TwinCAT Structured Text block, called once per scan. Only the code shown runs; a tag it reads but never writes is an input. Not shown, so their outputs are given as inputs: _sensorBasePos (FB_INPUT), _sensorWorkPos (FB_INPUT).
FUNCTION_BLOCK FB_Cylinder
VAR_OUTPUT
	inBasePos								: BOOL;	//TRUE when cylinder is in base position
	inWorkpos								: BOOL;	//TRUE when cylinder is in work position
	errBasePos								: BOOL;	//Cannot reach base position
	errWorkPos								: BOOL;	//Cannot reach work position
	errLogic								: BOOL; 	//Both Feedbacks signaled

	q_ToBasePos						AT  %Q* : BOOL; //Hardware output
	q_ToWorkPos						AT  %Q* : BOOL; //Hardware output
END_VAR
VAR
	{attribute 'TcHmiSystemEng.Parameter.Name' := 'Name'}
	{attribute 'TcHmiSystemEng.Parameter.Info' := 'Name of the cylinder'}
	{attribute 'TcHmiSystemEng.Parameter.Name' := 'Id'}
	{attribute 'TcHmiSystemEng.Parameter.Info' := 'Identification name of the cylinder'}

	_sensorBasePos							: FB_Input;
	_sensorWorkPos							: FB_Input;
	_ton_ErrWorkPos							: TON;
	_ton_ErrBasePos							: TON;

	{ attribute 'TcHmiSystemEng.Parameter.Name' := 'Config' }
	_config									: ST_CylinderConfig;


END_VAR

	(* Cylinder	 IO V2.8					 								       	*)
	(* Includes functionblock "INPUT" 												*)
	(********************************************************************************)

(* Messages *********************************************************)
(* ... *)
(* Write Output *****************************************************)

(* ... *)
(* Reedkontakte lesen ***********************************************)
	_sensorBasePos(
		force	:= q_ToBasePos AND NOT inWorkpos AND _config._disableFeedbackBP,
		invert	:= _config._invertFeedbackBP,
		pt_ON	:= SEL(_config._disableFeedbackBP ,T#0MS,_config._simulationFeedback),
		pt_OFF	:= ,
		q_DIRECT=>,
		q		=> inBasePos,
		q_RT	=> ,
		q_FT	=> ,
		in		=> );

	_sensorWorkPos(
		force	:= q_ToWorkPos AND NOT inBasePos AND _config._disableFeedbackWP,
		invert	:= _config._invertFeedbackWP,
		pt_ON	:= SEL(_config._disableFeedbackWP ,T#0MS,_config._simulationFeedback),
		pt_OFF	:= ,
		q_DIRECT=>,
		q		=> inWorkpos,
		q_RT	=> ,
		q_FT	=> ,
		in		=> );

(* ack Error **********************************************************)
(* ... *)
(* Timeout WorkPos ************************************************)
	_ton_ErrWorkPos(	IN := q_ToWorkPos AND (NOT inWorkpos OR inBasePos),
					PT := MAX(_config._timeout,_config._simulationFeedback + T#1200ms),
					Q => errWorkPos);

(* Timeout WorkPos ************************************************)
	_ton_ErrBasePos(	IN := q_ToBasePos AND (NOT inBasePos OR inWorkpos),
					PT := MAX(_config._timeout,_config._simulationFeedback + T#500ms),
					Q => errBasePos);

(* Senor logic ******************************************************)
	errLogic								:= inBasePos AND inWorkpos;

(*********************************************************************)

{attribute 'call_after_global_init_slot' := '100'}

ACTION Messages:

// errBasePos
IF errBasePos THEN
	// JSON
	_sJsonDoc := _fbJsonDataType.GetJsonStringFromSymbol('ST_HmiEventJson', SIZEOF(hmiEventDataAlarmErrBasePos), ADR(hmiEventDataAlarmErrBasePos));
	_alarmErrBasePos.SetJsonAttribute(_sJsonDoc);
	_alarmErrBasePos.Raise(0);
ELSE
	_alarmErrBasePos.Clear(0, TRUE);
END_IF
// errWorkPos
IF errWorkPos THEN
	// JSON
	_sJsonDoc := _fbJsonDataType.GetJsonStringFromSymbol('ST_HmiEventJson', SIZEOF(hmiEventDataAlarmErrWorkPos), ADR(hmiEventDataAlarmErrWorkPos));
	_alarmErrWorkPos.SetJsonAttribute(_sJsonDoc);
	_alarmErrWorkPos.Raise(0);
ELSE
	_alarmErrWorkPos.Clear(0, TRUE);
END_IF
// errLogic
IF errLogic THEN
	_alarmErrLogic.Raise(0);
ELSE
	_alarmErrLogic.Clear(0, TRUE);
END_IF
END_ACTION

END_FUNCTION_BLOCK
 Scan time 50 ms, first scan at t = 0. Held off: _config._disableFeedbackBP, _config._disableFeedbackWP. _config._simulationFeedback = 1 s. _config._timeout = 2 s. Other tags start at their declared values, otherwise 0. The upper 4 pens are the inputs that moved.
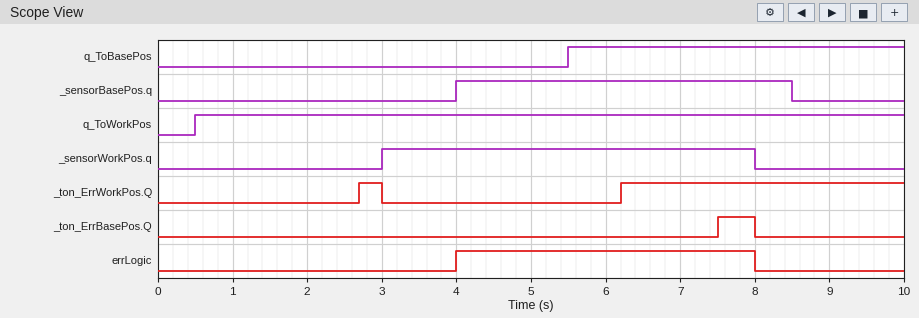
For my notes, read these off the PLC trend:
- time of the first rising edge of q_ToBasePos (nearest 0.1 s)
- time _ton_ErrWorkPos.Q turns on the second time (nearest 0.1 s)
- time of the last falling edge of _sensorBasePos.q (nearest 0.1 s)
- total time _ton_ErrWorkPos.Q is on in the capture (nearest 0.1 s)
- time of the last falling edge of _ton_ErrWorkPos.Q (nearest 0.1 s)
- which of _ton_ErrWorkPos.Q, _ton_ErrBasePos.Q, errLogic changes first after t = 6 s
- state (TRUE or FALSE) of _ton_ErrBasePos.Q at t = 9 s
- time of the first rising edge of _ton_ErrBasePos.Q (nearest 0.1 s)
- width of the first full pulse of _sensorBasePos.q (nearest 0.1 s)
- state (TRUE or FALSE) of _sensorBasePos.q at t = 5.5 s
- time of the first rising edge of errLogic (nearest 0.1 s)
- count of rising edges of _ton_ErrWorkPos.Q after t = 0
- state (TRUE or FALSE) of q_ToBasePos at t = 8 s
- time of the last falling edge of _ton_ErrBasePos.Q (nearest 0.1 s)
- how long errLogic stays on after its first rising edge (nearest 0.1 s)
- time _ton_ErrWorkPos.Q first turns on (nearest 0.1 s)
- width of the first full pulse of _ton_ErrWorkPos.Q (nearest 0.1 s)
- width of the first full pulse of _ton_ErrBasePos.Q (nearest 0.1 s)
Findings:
5.5 s
6.2 s
8.5 s
4.1 s
3.0 s
_ton_ErrWorkPos.Q
FALSE
7.5 s
4.5 s
TRUE
4.0 s
2
TRUE
8.0 s
4.0 s
2.7 s
0.3 s
0.5 s
